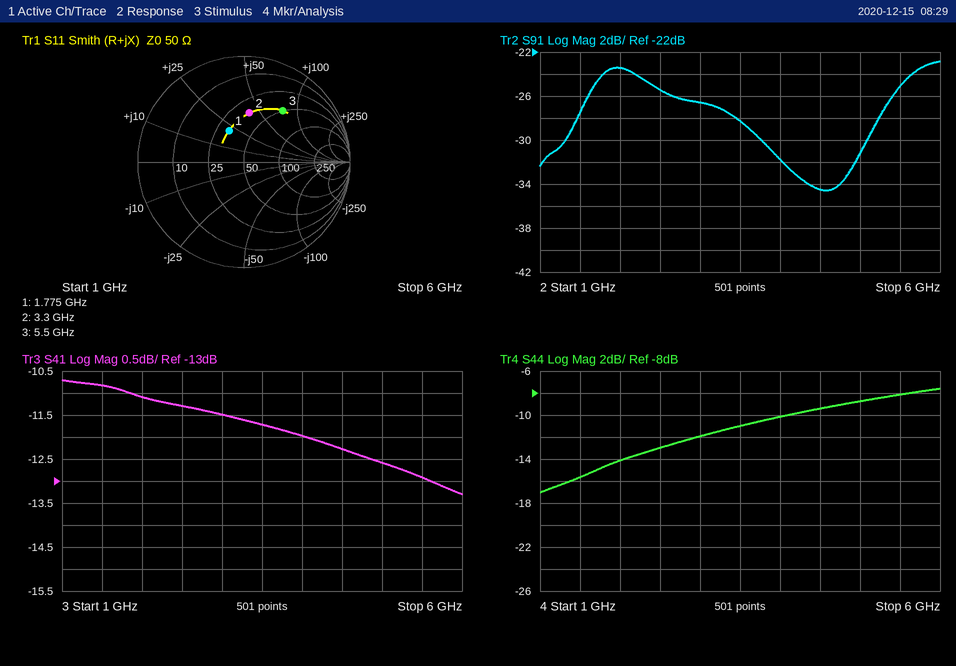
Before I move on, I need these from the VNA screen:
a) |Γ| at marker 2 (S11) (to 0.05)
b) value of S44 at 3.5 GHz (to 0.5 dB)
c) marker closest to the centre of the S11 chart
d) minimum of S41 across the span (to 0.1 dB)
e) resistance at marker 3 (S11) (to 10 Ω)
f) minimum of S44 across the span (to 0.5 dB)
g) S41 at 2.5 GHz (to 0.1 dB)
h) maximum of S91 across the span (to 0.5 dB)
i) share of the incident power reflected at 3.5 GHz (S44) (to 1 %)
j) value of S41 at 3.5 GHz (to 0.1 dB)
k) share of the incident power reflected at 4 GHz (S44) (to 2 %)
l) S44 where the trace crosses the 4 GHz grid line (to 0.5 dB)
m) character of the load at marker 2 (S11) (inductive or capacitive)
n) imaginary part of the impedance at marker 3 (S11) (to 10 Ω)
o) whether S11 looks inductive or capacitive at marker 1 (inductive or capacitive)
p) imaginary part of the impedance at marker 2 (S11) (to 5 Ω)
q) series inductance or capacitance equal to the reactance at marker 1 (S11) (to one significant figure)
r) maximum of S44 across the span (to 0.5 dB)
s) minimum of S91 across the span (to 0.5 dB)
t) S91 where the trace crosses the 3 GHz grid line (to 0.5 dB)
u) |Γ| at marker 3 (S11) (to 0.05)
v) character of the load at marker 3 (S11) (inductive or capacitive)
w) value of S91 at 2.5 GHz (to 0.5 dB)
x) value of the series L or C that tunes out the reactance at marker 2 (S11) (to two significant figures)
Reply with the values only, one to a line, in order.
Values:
0.45
-11.0 dB
marker 1
-13.3 dB
50 Ω
-17.0 dB
-11.3 dB
-23.0 dB
8 %
-11.7 dB
10 %
-10.0 dB
inductive
+80 Ω
inductive
+40 Ω
2 nH
-7.5 dB
-34.5 dB
-26.5 dB
0.60
inductive
-25.5 dB
1.2 pF
